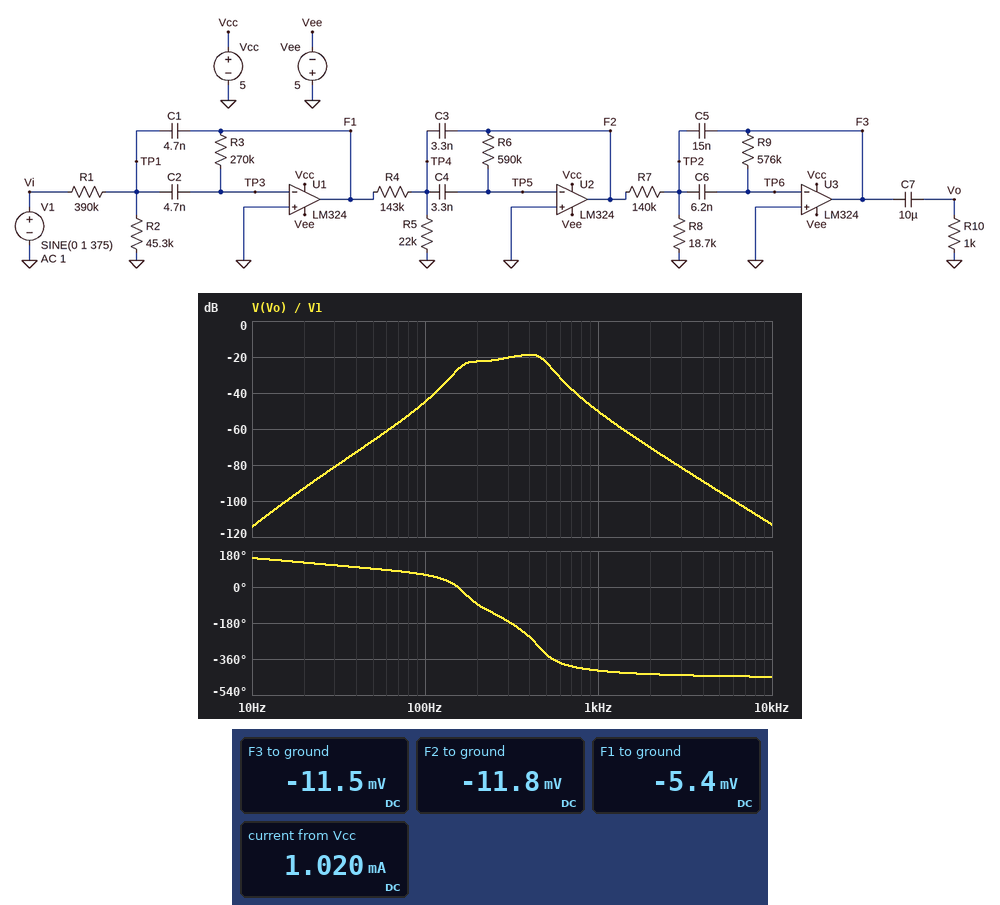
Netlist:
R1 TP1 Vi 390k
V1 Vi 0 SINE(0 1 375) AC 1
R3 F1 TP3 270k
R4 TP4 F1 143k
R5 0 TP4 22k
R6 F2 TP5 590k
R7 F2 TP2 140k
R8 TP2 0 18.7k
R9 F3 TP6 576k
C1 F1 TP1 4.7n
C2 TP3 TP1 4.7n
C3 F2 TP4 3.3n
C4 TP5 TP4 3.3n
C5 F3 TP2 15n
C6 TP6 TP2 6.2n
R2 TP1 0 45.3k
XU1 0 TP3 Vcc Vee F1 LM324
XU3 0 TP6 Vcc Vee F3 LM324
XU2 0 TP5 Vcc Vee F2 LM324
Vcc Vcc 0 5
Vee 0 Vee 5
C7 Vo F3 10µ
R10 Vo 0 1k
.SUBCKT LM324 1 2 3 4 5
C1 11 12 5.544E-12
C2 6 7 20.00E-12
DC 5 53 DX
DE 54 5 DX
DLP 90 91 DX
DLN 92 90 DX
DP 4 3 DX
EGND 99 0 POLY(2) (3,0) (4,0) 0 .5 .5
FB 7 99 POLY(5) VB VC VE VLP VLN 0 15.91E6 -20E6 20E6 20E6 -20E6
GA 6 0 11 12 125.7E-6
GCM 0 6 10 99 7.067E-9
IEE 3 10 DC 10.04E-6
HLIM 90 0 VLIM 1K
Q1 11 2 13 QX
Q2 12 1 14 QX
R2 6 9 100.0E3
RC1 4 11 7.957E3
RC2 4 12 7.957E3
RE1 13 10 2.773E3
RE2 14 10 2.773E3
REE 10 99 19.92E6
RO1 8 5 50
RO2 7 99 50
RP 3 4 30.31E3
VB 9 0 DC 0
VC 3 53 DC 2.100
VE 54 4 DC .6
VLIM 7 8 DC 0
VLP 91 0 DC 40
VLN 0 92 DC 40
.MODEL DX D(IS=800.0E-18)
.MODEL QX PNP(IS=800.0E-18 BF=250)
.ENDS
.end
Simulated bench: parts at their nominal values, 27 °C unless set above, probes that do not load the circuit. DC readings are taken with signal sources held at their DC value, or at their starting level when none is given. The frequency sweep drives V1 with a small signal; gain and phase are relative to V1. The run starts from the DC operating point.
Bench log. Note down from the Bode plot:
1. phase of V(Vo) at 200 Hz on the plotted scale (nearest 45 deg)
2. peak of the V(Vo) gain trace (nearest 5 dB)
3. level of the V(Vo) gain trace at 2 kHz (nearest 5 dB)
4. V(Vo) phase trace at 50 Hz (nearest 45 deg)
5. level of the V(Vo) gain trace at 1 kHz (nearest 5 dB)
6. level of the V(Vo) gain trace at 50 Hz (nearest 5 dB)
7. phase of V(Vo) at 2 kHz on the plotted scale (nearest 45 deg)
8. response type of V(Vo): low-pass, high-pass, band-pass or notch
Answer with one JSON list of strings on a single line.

["-90 deg", "-20 dB", "-70 dB", "90 deg", "-50 dB", "-65 dB", "-450 deg", "band-pass"]
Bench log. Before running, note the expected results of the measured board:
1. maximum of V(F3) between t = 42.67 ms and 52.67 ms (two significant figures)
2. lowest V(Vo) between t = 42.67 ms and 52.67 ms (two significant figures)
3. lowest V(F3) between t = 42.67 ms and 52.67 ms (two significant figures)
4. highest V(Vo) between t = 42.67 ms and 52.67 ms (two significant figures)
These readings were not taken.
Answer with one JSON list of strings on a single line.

["100 mV", "-110 mV", "-120 mV", "110 mV"]
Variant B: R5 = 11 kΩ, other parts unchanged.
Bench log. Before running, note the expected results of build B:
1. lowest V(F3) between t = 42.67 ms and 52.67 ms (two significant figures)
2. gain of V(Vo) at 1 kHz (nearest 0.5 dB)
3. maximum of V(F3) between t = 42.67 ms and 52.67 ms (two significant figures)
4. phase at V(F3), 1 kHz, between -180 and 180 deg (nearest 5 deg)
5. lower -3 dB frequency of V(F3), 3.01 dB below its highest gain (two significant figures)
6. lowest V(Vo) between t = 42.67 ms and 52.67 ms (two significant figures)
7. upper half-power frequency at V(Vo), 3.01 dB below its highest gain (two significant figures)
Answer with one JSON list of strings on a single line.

["-52 mV", "-48.5 dB", "29 mV", "-55 deg", "170 Hz", "-40 mV", "660 Hz"]
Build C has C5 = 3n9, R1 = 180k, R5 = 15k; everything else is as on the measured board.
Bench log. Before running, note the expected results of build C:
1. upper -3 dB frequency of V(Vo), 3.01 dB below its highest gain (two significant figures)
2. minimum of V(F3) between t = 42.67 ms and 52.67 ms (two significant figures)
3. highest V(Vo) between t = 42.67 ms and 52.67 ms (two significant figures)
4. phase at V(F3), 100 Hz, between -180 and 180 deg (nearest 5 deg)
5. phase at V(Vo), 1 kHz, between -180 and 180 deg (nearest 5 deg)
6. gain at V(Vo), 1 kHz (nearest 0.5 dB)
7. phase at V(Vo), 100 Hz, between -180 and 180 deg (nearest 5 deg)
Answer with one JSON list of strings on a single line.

["520 Hz", "-1.2 V", "1.2 V", "65 deg", "-55 deg", "-30.5 dB", "75 deg"]
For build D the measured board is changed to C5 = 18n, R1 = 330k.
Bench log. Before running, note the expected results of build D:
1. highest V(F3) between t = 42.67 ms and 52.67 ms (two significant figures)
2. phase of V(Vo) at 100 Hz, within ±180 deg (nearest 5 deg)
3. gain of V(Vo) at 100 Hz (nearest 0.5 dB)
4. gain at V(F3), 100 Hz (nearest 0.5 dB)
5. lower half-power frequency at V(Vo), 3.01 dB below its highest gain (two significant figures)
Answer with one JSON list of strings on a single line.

["96 mV", "55 deg", "-43.0 dB", "-42.5 dB", "270 Hz"]
